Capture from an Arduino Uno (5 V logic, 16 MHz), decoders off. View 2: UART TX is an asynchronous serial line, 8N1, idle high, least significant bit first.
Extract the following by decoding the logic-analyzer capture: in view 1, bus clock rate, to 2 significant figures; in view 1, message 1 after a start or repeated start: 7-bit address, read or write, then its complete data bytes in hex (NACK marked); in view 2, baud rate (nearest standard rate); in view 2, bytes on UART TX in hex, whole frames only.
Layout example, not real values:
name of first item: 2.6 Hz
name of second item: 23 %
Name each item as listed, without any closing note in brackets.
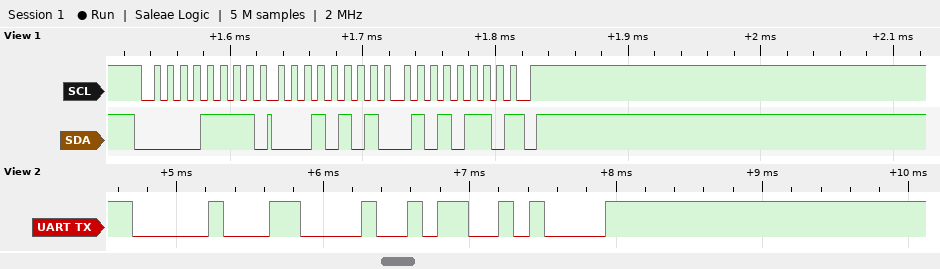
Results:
in view 1, bus clock rate, to 2 significant figures: 100 kHz
in view 1, message 1 after a start or repeated start: 7-bit address, read or write, then its complete data bytes in hex: 0x07 read: 15 56 NACK
in view 2, baud rate: 9600 baud
in view 2, bytes on UART TX in hex, whole frames only: 10 48 0A
